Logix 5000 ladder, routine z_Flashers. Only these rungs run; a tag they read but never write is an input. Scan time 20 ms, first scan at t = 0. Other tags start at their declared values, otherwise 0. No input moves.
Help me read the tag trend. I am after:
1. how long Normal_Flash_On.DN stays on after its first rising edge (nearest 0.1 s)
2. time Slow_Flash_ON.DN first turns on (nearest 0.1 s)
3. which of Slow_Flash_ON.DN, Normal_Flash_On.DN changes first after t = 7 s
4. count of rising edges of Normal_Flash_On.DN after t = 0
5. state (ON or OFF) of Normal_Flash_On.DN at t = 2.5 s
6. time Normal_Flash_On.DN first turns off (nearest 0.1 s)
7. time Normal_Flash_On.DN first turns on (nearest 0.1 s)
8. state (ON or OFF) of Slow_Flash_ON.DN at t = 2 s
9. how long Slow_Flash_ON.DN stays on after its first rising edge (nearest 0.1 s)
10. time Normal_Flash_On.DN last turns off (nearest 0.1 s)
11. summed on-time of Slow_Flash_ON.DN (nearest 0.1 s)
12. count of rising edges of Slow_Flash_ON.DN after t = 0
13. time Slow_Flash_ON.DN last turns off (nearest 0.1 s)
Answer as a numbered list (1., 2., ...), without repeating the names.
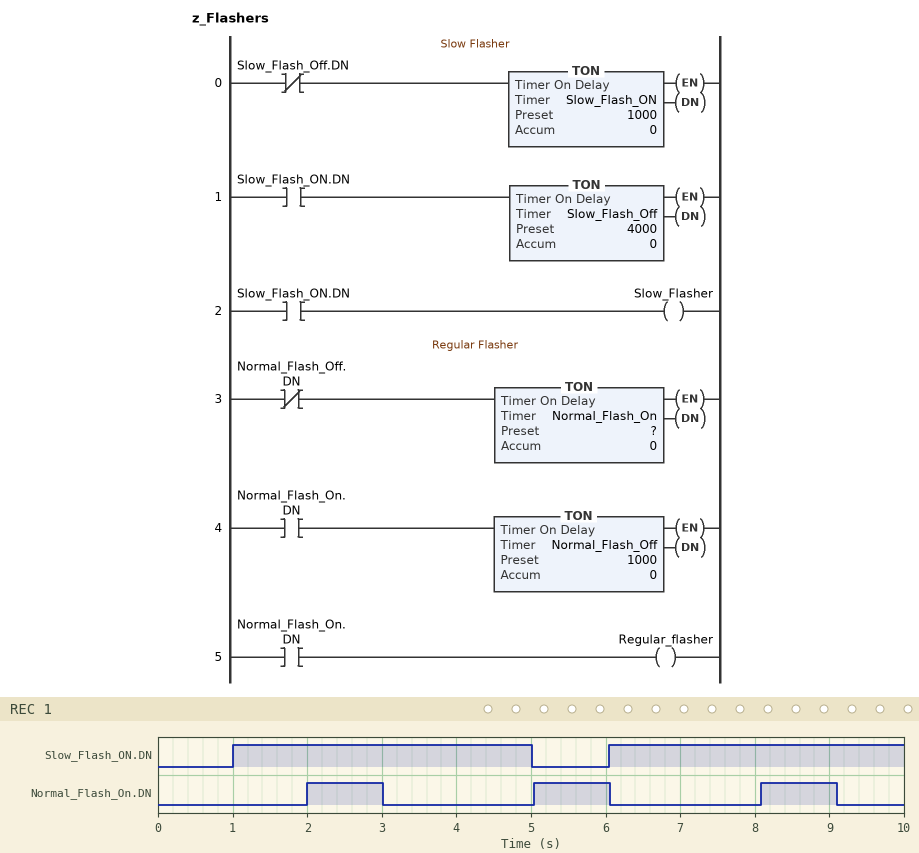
1. 1.0 s
2. 1.0 s
3. Normal_Flash_On.DN
4. 3
5. ON
6. 3.0 s
7. 2.0 s
8. ON
9. 4.0 s
10. 9.1 s
11. 8.0 s
12. 2
13. 5.0 s
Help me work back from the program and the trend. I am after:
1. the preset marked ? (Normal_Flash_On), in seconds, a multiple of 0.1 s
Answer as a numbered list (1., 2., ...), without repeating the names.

1. 2.0 s
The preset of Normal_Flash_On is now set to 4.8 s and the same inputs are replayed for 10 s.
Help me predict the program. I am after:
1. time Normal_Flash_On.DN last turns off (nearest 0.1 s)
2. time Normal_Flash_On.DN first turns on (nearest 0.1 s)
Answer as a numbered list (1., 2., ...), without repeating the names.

1. 5.8 s
2. 4.8 s
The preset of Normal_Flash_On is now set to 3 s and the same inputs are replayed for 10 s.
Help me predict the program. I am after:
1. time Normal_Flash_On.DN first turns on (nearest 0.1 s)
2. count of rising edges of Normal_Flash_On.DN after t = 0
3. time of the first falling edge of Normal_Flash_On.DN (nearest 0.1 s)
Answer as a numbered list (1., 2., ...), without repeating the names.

1. 3.0 s
2. 2
3. 4.0 s
